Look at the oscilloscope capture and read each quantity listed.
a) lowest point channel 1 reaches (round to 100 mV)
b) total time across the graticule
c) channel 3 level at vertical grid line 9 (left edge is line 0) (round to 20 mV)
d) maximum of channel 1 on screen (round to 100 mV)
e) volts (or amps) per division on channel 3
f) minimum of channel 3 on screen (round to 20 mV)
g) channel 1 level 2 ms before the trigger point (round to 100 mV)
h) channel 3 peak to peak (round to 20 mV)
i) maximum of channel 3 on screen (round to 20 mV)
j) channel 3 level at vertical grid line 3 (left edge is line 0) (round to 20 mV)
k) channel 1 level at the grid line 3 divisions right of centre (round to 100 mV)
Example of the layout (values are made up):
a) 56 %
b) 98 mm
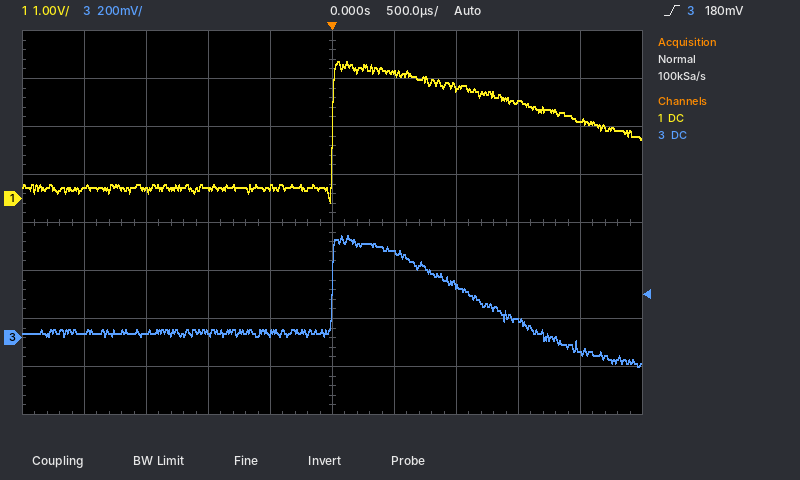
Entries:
a) -100 mV
b) 5 ms
c) -60 mV
d) 2.9 V
e) 200 mV
f) -120 mV
g) 200 mV
h) 540 mV
i) 420 mV
j) 20 mV
k) 2.0 V
